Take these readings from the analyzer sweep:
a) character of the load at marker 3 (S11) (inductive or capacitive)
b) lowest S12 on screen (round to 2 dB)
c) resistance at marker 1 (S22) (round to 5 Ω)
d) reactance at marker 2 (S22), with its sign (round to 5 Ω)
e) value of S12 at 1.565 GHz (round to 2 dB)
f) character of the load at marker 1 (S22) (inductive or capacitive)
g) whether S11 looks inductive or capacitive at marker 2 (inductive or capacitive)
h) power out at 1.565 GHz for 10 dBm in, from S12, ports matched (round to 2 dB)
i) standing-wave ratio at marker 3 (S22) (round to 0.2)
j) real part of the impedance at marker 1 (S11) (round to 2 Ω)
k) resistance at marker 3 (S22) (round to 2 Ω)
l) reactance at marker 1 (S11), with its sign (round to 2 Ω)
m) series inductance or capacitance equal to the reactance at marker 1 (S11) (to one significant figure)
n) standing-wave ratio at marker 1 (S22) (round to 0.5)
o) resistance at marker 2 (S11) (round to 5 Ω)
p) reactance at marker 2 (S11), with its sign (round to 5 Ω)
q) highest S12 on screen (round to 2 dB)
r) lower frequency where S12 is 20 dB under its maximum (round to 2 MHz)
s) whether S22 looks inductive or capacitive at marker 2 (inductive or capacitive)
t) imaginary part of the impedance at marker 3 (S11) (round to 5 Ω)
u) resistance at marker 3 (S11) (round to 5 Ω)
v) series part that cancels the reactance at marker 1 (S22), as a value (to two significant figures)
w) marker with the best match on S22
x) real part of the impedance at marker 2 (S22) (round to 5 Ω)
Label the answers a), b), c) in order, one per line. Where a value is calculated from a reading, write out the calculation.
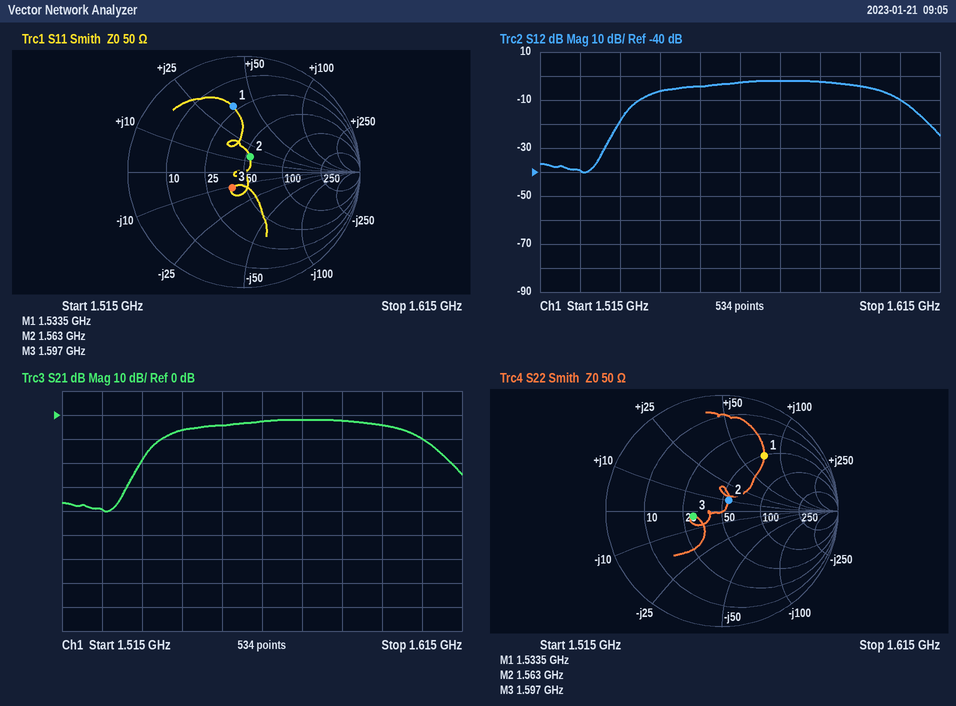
a) capacitive
b) -40 dB
c) 50 Ω
d) +10 Ω
e) -2 dB
f) inductive
g) inductive
h) 10 dBm + (-2 dB) = 8 dBm
i) 1.6
j) 22 Ω
k) 30 Ω
l) +38 Ω
m) L = 38 Ω/(2π × 1.5335 GHz) ≈ 4 nH
n) 4.0
o) 55 Ω
p) +15 Ω
q) -2 dB
r) 1.534 GHz
s) inductive
t) -10 Ω
u) 40 Ω
v) C = 1/(2π × 1.5335 GHz × 75 Ω) ≈ 1.4 pF
w) marker 2
x) 55 Ω
